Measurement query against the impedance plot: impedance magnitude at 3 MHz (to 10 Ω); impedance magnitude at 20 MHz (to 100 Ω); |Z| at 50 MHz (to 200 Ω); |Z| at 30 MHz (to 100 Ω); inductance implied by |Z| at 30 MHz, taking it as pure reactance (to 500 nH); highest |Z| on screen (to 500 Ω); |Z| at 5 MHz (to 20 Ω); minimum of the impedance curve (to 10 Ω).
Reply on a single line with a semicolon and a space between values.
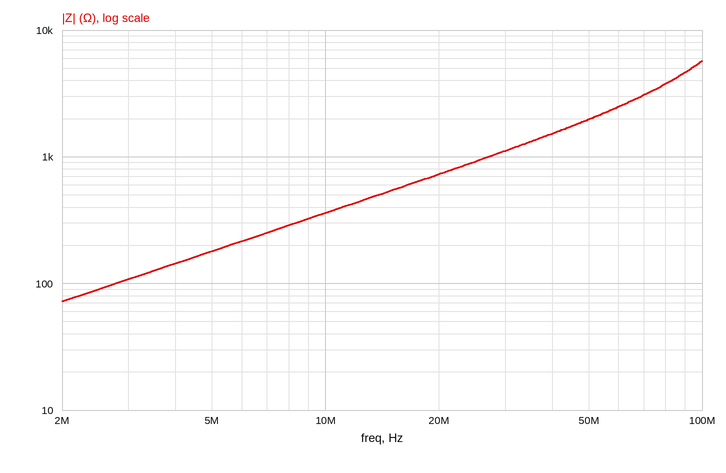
110 Ω; 700 Ω; 2.0 kΩ; 1.1 kΩ; 6.0 µH; 5.5 kΩ; 180 Ω; 70 Ω
